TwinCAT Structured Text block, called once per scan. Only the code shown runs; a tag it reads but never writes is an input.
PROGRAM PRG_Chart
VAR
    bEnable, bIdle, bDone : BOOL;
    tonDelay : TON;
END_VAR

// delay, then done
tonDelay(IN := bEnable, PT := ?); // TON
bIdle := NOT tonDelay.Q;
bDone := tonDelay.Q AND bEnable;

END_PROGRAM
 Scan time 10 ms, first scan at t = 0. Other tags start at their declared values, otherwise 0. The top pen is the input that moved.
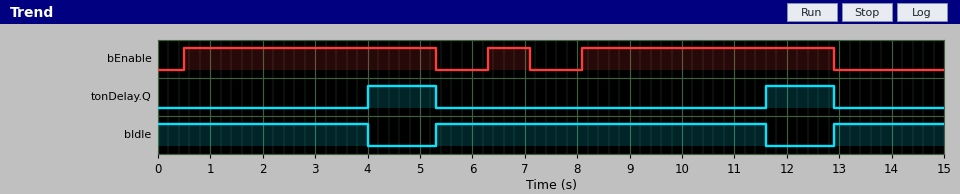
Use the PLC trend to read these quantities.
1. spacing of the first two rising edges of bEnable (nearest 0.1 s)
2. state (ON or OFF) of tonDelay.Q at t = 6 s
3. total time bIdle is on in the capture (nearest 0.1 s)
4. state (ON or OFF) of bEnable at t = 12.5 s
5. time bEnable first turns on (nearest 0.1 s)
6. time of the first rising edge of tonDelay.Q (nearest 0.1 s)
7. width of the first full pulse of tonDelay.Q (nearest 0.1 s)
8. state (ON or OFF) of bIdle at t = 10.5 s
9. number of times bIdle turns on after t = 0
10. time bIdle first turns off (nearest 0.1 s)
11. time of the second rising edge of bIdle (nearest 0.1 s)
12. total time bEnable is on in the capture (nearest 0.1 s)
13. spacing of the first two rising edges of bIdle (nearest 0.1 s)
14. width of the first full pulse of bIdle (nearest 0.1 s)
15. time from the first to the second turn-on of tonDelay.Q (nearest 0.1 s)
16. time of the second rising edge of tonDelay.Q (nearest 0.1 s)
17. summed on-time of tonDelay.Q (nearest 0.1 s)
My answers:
5.8 s
OFF
12.4 s
ON
0.5 s
4.0 s
1.3 s
ON
2
4.0 s
12.9 s
10.4 s
7.6 s
6.3 s
7.6 s
11.6 s
2.6 s
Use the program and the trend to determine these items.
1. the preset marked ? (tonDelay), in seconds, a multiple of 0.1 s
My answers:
3.5 s
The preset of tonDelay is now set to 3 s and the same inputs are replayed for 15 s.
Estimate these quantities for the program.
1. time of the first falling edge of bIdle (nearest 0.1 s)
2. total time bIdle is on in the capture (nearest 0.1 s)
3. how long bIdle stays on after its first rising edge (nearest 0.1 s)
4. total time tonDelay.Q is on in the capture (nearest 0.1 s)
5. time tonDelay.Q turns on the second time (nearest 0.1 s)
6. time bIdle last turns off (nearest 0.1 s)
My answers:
3.5 s
11.4 s
5.8 s
3.6 s
11.1 s
11.1 s
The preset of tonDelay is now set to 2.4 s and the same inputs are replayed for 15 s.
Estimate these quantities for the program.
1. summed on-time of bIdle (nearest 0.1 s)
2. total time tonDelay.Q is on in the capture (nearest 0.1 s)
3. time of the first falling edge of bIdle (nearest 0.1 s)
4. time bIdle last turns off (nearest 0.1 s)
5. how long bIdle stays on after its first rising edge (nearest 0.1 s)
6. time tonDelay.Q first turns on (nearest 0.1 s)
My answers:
10.2 s
4.8 s
2.9 s
10.5 s
5.2 s
2.9 s
